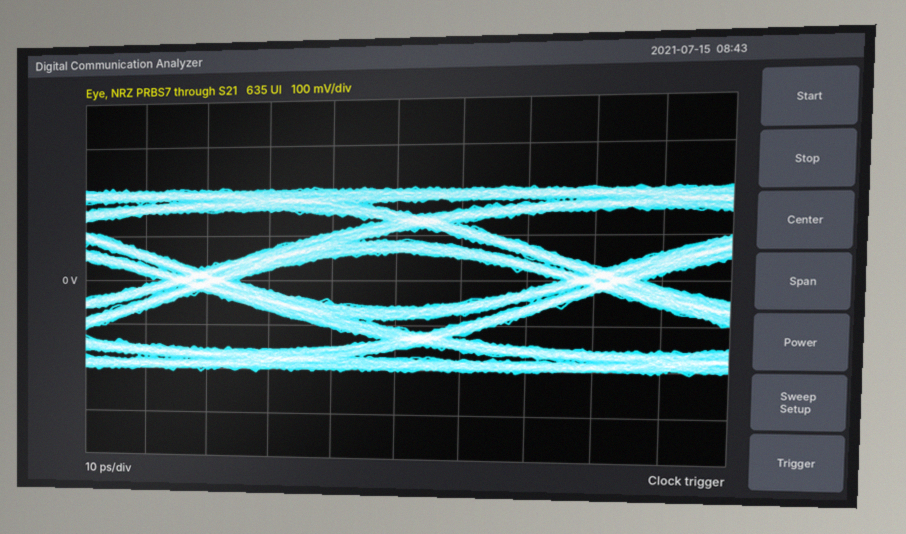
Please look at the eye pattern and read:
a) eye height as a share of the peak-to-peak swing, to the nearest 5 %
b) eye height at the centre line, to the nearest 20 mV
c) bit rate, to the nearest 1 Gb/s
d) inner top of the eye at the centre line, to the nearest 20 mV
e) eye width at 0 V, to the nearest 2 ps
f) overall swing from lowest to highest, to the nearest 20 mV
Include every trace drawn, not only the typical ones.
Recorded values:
30 %
120 mV
16 Gb/s
60 mV
50 ps
420 mV
